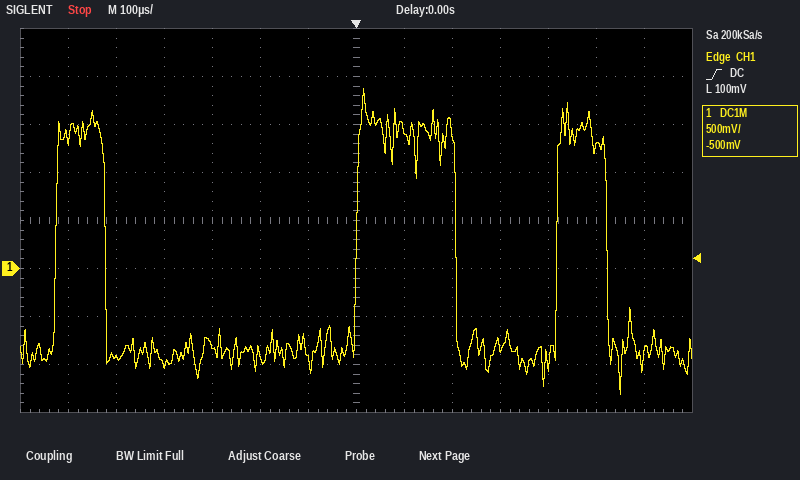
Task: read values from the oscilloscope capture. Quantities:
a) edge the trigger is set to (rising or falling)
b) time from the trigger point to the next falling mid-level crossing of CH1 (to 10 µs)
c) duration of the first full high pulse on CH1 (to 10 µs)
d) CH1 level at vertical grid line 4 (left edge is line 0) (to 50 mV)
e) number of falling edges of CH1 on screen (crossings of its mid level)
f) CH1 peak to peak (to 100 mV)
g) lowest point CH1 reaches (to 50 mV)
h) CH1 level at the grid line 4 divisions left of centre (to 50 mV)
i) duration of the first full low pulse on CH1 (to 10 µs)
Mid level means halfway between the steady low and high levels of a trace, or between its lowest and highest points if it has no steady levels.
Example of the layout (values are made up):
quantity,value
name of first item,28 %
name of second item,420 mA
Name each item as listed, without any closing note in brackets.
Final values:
quantity,value
edge the trigger is set to,rising
time from the trigger point to the next falling mid-level crossing of CH1,210 µs
duration of the first full high pulse on CH1,100 µs
CH1 level at vertical grid line 4 (left edge is line 0),-800 mV
number of falling edges of CH1 on screen,3
CH1 peak to peak,3.20 V
lowest point CH1 reaches,-1.30 V
CH1 level at the grid line 4 divisions left of centre,-1.00 V
duration of the first full low pulse on CH1,520 µs
